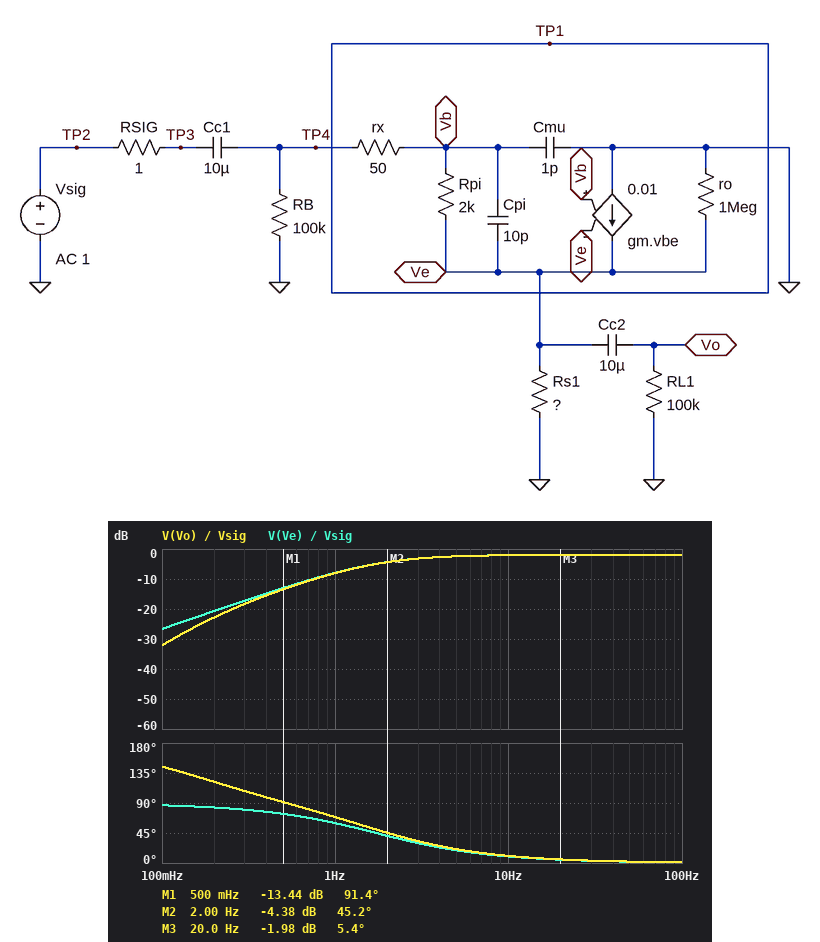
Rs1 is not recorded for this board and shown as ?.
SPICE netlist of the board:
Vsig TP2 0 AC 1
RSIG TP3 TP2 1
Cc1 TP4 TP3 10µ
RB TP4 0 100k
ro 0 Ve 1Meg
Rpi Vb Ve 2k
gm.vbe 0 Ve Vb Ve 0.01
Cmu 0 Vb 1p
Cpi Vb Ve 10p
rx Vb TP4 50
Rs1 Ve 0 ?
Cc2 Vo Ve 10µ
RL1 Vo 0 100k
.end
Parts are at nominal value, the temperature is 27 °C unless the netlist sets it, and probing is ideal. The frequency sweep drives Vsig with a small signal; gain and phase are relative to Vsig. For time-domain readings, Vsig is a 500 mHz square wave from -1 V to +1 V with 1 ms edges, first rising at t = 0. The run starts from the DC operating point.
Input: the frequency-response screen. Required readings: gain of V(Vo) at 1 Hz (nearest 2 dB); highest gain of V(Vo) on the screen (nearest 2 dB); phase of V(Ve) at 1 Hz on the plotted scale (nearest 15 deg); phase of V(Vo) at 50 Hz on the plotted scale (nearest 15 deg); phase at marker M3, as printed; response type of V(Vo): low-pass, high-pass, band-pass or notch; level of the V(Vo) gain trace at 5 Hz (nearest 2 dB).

-8 dB
-2 dB
60 deg
0 deg
5.4 deg
high-pass
-2 dB
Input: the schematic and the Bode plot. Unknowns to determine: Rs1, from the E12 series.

390 Ω
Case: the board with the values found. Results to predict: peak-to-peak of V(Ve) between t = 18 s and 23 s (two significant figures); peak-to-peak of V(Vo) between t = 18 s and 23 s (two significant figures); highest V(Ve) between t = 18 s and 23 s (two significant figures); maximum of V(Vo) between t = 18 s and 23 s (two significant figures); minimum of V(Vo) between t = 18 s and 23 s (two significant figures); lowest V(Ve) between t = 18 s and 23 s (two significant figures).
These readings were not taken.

3.2 V
3.3 V
1.6 V
1.6 V
-1.6 V
-1.6 V
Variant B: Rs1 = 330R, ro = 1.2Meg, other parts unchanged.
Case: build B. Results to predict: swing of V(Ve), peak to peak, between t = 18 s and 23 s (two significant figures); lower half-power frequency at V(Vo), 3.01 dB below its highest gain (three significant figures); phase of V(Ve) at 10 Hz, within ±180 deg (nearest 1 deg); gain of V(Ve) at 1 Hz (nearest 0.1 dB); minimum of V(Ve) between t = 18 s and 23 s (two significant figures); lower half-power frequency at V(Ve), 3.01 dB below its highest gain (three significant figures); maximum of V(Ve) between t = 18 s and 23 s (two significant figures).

3.1 V
1.95 Hz
11 deg
-9.0 dB
-1.5 V
1.94 Hz
1.5 V
